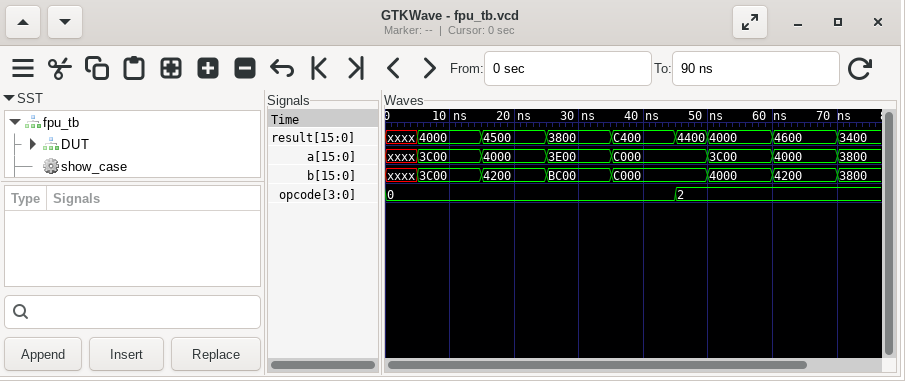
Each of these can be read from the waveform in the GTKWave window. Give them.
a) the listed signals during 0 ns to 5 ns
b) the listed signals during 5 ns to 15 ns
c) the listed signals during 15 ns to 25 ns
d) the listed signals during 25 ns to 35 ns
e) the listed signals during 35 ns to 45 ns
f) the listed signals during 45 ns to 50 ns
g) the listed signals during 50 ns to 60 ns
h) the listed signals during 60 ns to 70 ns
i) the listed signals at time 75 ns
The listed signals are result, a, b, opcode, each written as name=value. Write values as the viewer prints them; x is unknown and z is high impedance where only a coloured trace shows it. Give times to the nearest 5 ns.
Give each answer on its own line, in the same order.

result=xxxx, a=xxxx, b=xxxx, opcode=0
result=4000, a=3C00, b=3C00, opcode=0
result=4500, a=4000, b=4200, opcode=0
result=3800, a=3E00, b=BC00, opcode=0
result=C400, a=C000, b=C000, opcode=0
result=4400, a=C000, b=C000, opcode=2
result=4000, a=3C00, b=4000, opcode=2
result=4600, a=4000, b=4200, opcode=2
result=3400, a=3800, b=3800, opcode=2
